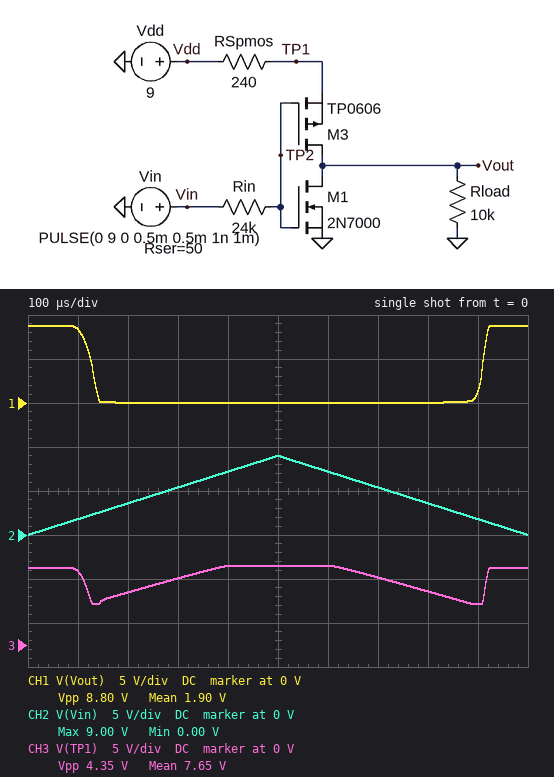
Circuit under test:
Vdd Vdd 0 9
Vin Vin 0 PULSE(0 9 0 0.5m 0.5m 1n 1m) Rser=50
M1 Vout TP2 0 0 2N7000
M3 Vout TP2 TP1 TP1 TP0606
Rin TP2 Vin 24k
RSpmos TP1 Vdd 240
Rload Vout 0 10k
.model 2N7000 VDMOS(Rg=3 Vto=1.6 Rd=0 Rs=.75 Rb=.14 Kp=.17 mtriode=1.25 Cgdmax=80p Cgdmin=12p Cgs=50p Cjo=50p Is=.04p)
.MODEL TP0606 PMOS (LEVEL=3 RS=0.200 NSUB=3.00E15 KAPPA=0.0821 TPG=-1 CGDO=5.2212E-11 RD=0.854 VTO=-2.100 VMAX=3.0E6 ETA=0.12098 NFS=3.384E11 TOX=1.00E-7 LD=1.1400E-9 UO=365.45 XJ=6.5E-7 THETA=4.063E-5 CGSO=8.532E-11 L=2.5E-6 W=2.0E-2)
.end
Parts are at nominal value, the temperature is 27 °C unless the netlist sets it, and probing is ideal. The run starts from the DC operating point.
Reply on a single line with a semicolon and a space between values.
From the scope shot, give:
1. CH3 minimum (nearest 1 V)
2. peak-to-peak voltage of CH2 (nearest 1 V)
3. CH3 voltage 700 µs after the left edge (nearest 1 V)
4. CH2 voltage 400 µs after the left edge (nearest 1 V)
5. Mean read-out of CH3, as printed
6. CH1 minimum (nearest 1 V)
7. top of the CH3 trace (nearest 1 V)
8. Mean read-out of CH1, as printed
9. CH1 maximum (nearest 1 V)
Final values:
5 V; 9 V; 8 V; 7 V; 7.65 V; 0 V; 9 V; 1.90 V; 9 V
